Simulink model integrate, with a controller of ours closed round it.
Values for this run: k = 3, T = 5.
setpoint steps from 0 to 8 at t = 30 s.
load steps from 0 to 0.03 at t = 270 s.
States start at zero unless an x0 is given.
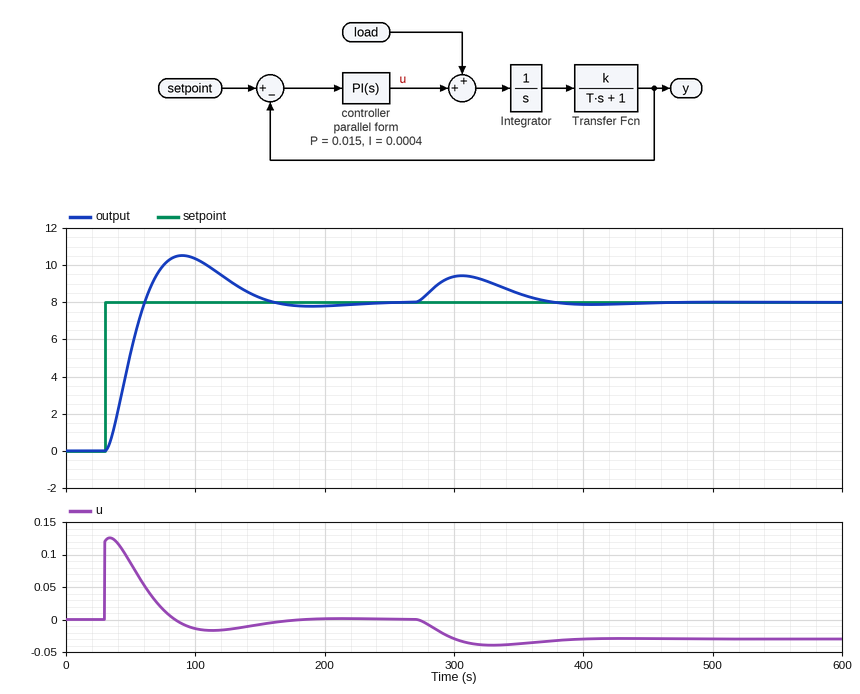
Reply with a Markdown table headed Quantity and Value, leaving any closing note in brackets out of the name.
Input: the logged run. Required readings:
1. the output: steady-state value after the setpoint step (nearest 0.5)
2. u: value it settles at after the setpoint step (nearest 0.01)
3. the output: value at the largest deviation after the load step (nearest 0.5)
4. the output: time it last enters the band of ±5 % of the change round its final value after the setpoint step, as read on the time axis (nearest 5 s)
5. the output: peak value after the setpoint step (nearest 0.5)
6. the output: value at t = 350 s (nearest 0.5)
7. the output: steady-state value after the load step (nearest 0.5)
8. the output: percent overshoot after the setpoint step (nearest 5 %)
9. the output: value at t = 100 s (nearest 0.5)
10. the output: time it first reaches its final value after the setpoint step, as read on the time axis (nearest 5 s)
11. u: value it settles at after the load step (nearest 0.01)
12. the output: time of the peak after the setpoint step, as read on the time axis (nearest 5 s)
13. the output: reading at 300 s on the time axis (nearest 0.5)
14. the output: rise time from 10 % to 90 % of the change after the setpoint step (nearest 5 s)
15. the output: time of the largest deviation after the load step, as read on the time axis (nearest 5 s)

| Quantity | Value |
|---|---|
| the output: steady-state value after the setpoint step | 8.0 |
| u: value it settles at after the setpoint step | 0.00 |
| the output: value at the largest deviation after the load step | 9.5 |
| the output: time it last enters the band of ±5 % of the change round its final value after the setpoint step, as read on the time axis | 145 s |
| the output: peak value after the setpoint step | 10.5 |
| the output: value at t = 350 s | 8.5 |
| the output: steady-state value after the load step | 8.0 |
| the output: percent overshoot after the setpoint step | 30 % |
| the output: value at t = 100 s | 10.5 |
| the output: time it first reaches its final value after the setpoint step, as read on the time axis | 60 s |
| u: value it settles at after the load step | -0.03 |
| the output: time of the peak after the setpoint step, as read on the time axis | 90 s |
| the output: reading at 300 s on the time axis | 9.5 |
| the output: rise time from 10 % to 90 % of the change after the setpoint step | 20 s |
| the output: time of the largest deviation after the load step, as read on the time axis | 305 s |
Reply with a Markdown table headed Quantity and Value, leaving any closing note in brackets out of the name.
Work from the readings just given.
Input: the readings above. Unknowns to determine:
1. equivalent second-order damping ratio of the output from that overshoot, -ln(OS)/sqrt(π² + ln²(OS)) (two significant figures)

| Quantity | Value |
|---|---|
| equivalent second-order damping ratio of the output from that overshoot, -ln(OS)/sqrt(π² + ln²(OS)) | 0.36 |
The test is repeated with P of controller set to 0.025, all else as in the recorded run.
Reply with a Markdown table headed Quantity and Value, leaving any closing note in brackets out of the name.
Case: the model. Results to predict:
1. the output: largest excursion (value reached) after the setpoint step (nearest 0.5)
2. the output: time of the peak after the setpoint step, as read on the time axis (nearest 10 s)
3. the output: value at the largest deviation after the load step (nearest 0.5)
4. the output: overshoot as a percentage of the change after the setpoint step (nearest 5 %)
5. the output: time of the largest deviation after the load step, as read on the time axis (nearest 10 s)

| Quantity | Value |
|---|---|
| the output: largest excursion (value reached) after the setpoint step | 9.5 |
| the output: time of the peak after the setpoint step, as read on the time axis | 70 s |
| the output: value at the largest deviation after the load step | 9.0 |
| the output: overshoot as a percentage of the change after the setpoint step | 20 % |
| the output: time of the largest deviation after the load step, as read on the time axis | 300 s |
